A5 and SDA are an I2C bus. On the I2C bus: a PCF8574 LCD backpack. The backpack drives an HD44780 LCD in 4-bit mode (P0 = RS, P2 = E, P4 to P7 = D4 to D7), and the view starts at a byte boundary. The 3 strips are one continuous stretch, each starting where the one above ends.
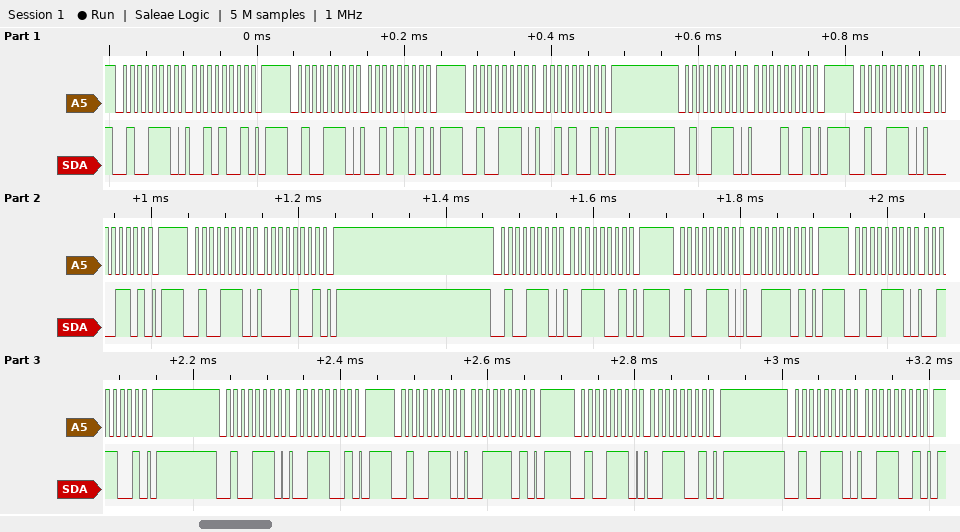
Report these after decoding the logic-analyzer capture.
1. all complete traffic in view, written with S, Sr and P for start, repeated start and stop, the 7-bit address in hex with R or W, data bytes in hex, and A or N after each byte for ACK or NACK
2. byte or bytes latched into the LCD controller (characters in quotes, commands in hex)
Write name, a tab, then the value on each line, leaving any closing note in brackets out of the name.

all complete traffic in view, written with S, Sr and P for start, repeated start and stop, the 7-bit address in hex with R or W, data bytes in hex, and A or N after each byte for ACK or NACK	S 27W A 29 A P S 27W A 2D A P S 27W A 29 A P S 27W A 09 A P S 27W A 0D A P S 27W A 09 A P S 27W A 39 A P S 27W A 3D A P S 27W A 39 A P S 27W A 39 A P S 27W A 3D A P S 27W A 39 A P S 27W A 39 A P
byte or bytes latched into the LCD controller	' ' '3'
